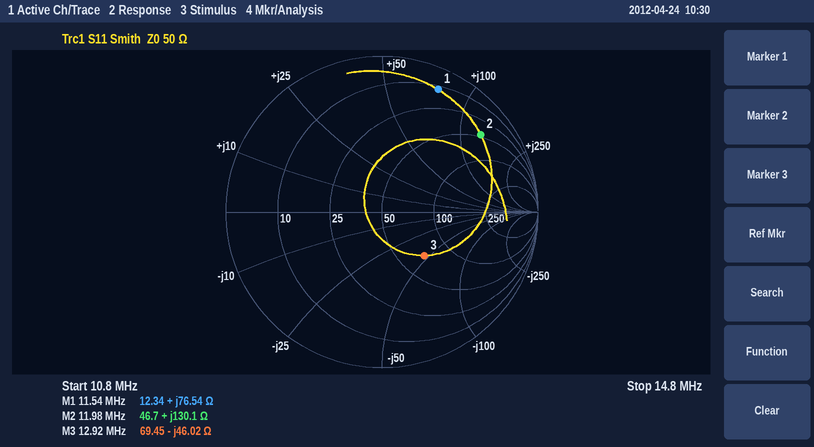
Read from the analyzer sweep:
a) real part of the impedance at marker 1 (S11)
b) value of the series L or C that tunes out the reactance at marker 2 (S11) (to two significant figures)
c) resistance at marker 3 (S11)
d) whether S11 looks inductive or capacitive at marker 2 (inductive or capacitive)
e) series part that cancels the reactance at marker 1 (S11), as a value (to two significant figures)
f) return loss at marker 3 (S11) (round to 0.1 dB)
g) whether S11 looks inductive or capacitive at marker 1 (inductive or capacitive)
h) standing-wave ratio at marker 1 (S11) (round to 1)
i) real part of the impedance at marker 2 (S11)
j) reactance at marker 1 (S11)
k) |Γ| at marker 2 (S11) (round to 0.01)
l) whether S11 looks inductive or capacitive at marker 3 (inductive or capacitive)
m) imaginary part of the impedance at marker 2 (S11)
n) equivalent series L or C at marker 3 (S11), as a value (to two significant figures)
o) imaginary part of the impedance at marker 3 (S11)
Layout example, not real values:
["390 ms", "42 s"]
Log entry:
["12.34 Ω", "100 pF", "69.45 Ω", "inductive", "180 pF", "8.2 dB", "inductive", "14", "46.7 Ω", "+76.54 Ω", "0.80", "capacitive", "+130.1 Ω", "270 pF", "-46.02 Ω"]
